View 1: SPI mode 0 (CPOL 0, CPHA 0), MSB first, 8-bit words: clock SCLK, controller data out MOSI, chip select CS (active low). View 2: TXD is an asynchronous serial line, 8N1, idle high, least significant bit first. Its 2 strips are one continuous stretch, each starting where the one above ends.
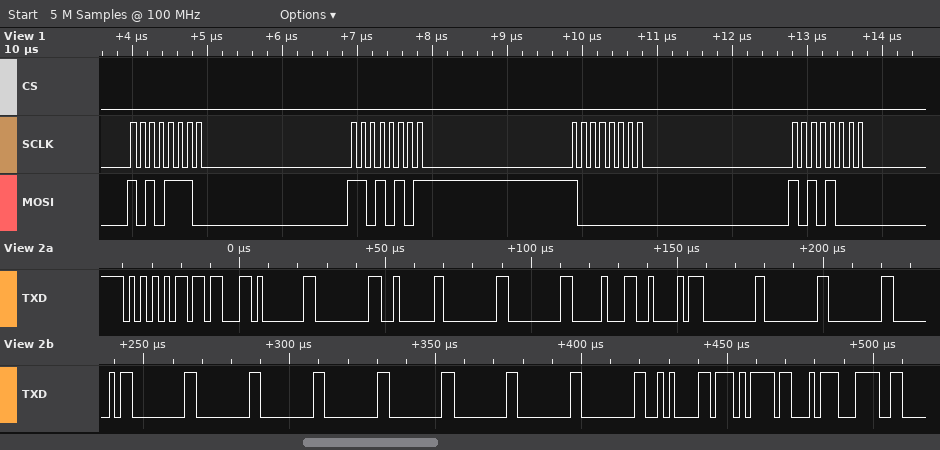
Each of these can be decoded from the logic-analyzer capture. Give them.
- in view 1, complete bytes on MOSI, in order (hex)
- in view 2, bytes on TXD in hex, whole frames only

AE D5 80 A8
0x55 0x1B 0x01 0x00 0x02 0x00 0x00 0x10 0x42 0x00 0x00 0x00 0x40 0x00 0x00 0x00 0x00 0x00 0x00 0x00 0x00 0x0A 0xD7 0xA3 0x3C
